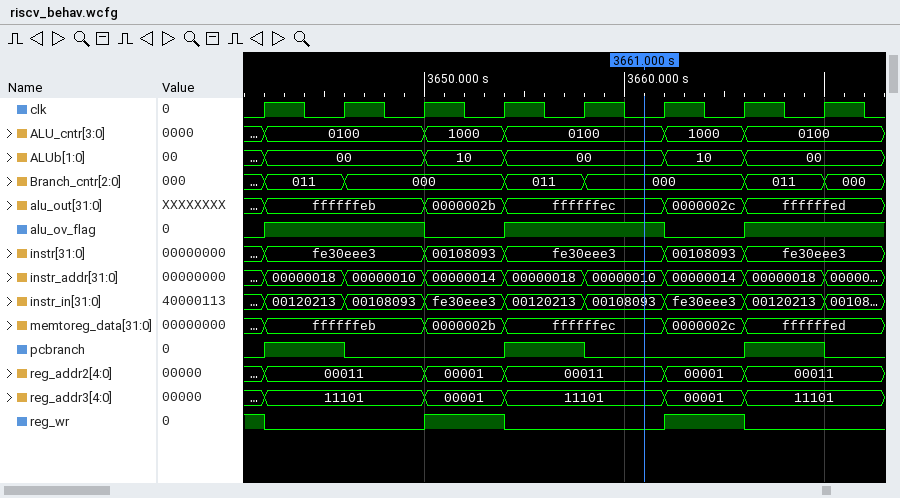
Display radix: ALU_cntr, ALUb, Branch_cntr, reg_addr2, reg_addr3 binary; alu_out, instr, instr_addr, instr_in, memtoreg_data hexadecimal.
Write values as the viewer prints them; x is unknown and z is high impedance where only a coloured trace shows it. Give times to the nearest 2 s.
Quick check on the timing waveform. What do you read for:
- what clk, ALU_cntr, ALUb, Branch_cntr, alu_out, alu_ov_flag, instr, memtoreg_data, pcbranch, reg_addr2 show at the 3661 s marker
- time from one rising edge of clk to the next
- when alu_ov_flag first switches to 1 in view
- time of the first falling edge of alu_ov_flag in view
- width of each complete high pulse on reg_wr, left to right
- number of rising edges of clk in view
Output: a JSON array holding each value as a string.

["clk=0, ALU_cntr=0100, ALUb=00, Branch_cntr=000, alu_out=ffffffec, alu_ov_flag=1, instr=fe30eee3, memtoreg_data=ffffffec, pcbranch=0, reg_addr2=00011", "4 s", "3642 s", "3650 s", "4 s, 4 s", "8"]
